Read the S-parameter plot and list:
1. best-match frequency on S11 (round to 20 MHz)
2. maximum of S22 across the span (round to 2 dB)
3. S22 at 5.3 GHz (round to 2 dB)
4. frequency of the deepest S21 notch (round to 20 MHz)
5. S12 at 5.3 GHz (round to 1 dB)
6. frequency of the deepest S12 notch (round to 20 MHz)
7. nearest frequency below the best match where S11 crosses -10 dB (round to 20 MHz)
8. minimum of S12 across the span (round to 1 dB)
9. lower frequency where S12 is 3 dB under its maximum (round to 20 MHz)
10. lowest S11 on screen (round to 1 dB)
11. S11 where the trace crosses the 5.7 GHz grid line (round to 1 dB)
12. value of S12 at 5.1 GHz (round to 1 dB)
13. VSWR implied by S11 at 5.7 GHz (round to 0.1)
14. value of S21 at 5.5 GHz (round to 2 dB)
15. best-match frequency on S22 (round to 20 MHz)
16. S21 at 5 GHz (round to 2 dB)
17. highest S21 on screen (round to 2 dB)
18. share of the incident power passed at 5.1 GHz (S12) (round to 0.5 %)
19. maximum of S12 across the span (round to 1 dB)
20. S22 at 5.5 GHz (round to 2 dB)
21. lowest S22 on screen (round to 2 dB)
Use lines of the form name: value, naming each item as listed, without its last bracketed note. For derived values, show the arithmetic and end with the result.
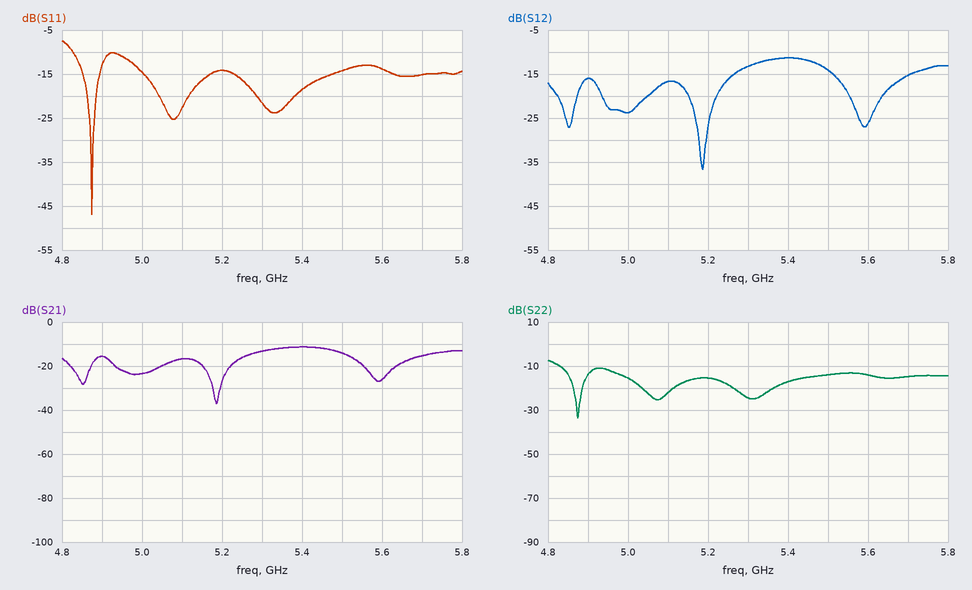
best-match frequency on S11: 4.88 GHz
maximum of S22 across the span: -8 dB
S22 at 5.3 GHz: -24 dB
frequency of the deepest S21 notch: 5.18 GHz
S12 at 5.3 GHz: -13 dB
frequency of the deepest S12 notch: 5.18 GHz
nearest frequency below the best match where S11 crosses -10 dB: 4.82 GHz
minimum of S12 across the span: -37 dB
lower frequency where S12 is 3 dB under its maximum: 5.28 GHz
lowest S11 on screen: -47 dB
S11 where the trace crosses the 5.7 GHz grid line: -15 dB
value of S12 at 5.1 GHz: -17 dB
VSWR implied by S11 at 5.7 GHz: |Γ| = 10^(-15/20) = 0.1778; VSWR = (1 + 0.1778)/(1 − 0.1778) ≈ 1.4
value of S21 at 5.5 GHz: -14 dB
best-match frequency on S22: 4.88 GHz
S21 at 5 GHz: -24 dB
highest S21 on screen: -12 dB
share of the incident power passed at 5.1 GHz (S12): 10^(-17/10) ≈ 2.0 %
maximum of S12 across the span: -11 dB
S22 at 5.5 GHz: -14 dB
lowest S22 on screen: -34 dB
